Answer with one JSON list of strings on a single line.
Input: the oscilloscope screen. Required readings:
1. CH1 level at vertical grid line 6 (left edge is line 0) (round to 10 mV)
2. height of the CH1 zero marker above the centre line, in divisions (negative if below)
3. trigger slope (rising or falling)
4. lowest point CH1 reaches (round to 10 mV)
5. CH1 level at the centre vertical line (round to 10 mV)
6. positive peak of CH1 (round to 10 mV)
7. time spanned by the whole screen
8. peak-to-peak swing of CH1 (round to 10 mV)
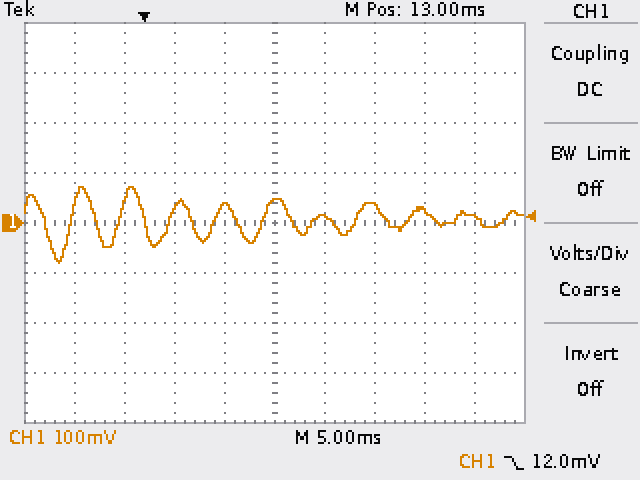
["10 mV", "0.0 div", "falling", "-80 mV", "40 mV", "70 mV", "50 ms", "150 mV"]
